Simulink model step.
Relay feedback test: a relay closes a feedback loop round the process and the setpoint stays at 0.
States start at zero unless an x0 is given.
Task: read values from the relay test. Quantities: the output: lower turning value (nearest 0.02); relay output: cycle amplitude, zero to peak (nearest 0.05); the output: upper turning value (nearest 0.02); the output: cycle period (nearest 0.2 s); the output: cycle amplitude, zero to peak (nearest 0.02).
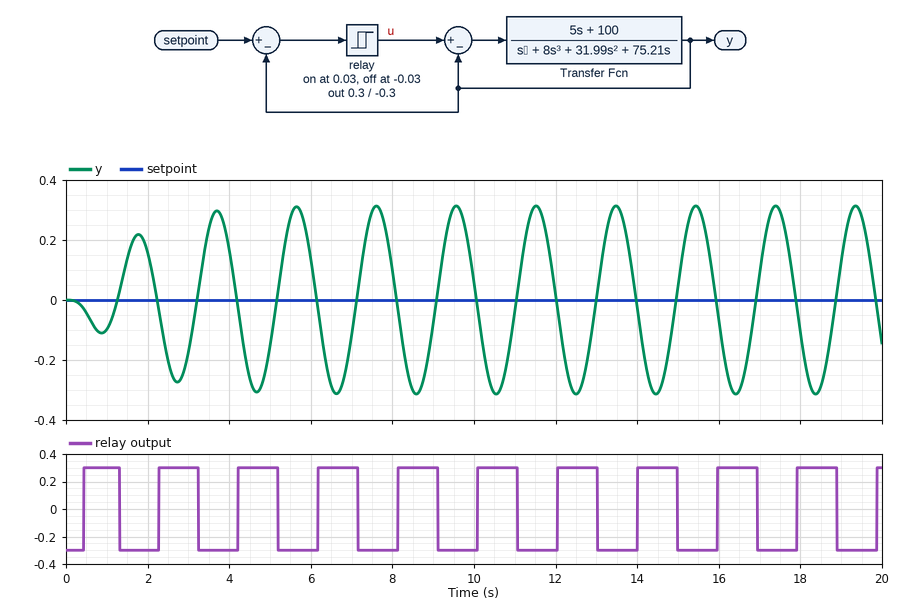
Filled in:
-0.32
0.30
0.32
2.0 s
0.32
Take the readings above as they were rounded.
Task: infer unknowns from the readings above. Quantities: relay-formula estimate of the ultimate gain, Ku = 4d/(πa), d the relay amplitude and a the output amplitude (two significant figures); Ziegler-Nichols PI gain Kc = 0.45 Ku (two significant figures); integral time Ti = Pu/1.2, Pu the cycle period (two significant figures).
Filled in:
1.2
0.54
1.7 s
